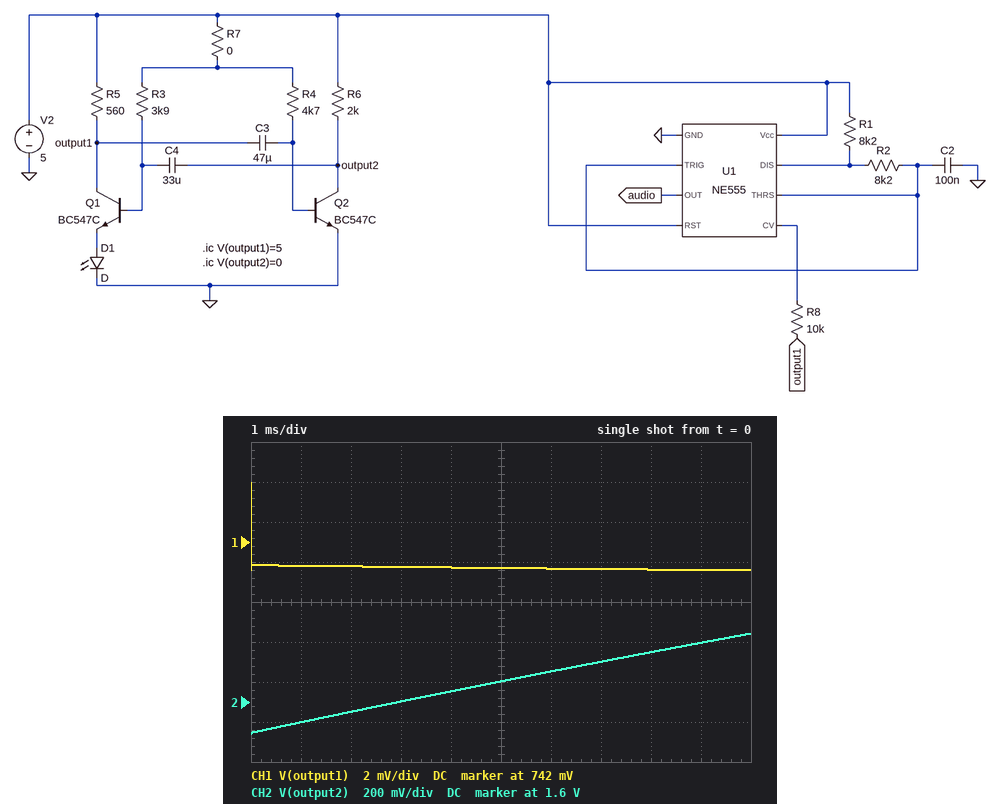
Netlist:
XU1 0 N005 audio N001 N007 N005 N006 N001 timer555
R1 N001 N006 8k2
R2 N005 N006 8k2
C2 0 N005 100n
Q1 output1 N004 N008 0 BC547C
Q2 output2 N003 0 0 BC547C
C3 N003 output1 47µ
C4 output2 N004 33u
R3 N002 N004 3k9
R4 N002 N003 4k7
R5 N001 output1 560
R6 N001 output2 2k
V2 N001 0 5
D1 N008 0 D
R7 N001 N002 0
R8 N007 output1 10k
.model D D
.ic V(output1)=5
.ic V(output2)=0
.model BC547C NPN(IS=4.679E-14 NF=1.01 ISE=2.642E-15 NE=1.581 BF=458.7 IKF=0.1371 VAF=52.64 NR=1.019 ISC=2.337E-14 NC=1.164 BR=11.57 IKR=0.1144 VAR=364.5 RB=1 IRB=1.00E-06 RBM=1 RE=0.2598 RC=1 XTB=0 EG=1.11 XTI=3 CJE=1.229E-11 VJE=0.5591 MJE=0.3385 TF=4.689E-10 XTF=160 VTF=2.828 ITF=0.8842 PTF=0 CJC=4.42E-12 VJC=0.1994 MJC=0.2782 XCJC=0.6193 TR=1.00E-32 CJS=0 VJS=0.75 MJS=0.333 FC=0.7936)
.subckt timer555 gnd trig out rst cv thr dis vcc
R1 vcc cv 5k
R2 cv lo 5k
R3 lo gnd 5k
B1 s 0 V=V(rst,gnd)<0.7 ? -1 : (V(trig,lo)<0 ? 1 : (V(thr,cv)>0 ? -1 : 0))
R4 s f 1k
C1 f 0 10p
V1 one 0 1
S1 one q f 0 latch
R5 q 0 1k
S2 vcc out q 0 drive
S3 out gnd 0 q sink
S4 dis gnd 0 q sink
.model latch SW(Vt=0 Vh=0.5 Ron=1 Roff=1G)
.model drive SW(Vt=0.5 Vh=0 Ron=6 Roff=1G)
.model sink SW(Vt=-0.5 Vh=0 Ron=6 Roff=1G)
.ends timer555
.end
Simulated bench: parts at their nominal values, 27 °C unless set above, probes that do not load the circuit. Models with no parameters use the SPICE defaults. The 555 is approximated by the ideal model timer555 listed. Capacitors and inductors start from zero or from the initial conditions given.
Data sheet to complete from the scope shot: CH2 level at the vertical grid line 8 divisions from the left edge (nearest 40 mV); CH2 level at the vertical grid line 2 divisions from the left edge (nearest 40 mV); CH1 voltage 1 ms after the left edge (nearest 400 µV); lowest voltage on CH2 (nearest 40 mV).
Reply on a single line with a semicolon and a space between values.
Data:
1.84 V; 1.56 V; 740.8 mV; 1.44 V
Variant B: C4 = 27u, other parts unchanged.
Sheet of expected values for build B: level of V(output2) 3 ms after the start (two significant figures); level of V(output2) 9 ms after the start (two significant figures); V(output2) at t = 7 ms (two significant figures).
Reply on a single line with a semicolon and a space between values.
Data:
1.6 V; 2.0 V; 1.9 V
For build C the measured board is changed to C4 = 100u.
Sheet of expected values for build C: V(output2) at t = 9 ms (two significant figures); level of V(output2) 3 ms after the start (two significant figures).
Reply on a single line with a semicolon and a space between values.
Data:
1.6 V; 1.5 V
